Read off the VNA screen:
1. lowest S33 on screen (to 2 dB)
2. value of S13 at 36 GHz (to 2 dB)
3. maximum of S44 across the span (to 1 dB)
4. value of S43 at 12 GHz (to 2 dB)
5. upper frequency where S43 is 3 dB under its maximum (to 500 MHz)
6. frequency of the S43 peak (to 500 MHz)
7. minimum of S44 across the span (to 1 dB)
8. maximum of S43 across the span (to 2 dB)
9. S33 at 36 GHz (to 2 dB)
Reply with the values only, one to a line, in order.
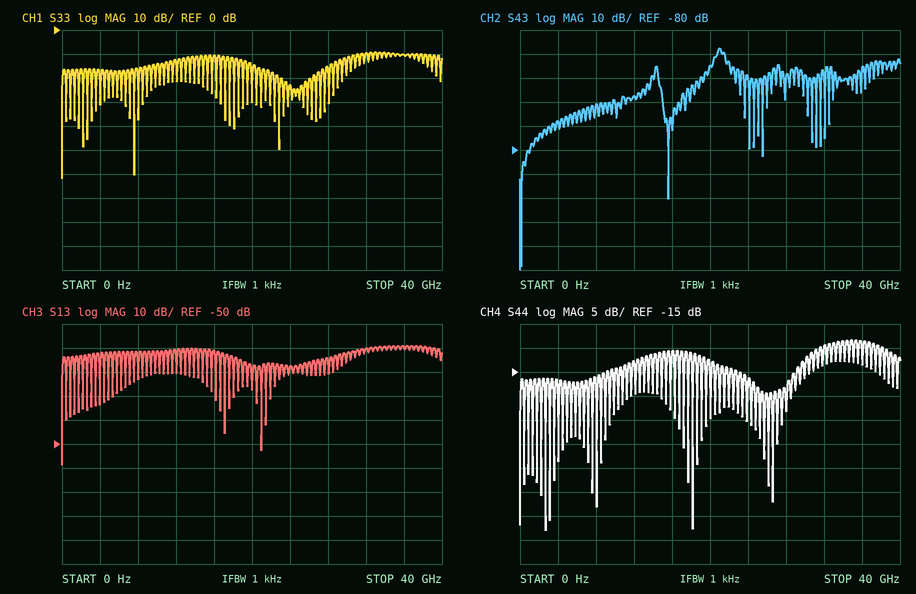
-62 dB
-10 dB
-8 dB
-58 dB
21.5 GHz
21.0 GHz
-48 dB
-38 dB
-10 dB
